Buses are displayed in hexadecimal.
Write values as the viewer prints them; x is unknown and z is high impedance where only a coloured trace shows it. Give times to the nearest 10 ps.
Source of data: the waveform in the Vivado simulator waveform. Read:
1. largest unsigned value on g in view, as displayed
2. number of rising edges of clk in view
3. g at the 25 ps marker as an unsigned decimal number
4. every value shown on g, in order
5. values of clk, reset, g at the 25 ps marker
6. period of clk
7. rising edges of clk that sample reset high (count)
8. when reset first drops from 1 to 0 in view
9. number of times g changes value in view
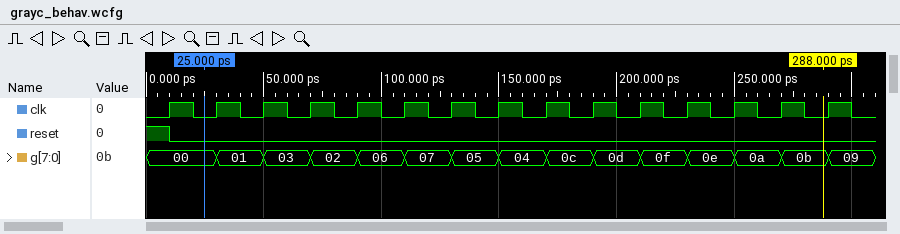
0f
15
0
00, 01, 03, 02, 06, 07, 05, 04, 0c, 0d, 0f, 0e, 0a, 0b, 09
clk=0, reset=0, g=00
20 ps
1
10 ps
14
